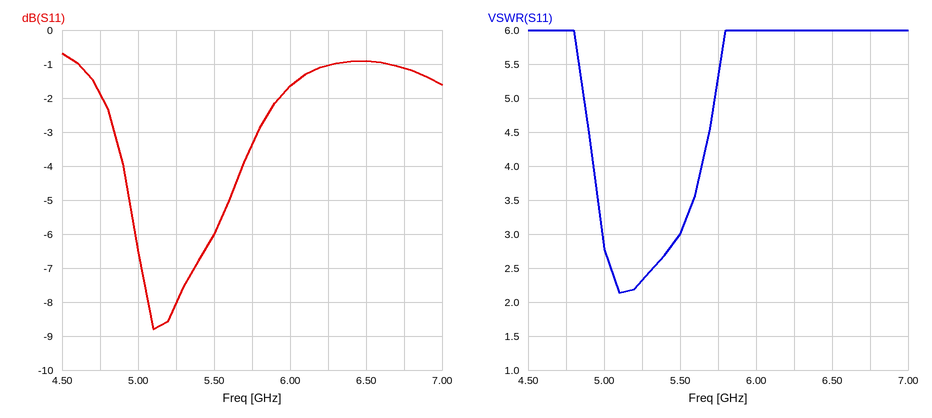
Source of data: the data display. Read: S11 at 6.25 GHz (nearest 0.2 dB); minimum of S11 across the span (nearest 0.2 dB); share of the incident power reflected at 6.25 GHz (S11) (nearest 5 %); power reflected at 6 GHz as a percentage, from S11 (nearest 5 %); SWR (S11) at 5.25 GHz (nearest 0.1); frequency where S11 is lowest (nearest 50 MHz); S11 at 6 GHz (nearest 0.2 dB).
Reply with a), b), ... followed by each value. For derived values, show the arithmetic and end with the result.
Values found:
a) -1.0 dB
b) -8.8 dB
c) 10^(-1/10) ≈ 79.4 %, so 80 % to the nearest 5 %
d) 10^(-1.6/10) ≈ 69.2 %, so 70 % to the nearest 5 %
e) 2.3
f) 5.10 GHz
g) -1.6 dB
